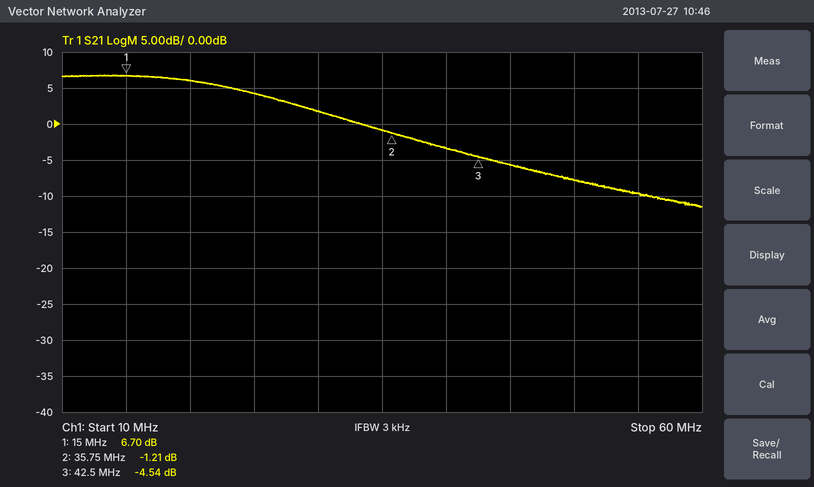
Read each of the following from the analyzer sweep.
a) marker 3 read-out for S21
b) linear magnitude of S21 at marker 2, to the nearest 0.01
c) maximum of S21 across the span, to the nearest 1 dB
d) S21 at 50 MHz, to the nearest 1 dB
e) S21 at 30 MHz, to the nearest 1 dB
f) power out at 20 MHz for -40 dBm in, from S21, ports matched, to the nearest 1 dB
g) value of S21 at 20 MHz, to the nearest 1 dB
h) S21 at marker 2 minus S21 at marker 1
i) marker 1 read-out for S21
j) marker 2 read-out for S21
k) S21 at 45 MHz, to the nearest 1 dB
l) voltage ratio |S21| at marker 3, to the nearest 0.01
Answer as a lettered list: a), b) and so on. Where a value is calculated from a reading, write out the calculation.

a) -4.54 dB
b) 10^(-1.21/20) ≈ 0.87
c) 7 dB
d) -8 dB
e) 2 dB
f) -40 dBm + (6 dB) = -34 dBm
g) 6 dB
h) -1.21 − (6.7) = -7.91 dB
i) 6.70 dB
j) -1.21 dB
k) -6 dB
l) 10^(-4.54/20) ≈ 0.59
